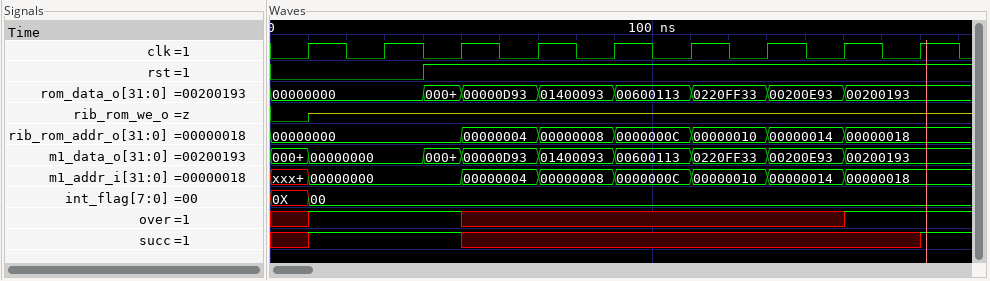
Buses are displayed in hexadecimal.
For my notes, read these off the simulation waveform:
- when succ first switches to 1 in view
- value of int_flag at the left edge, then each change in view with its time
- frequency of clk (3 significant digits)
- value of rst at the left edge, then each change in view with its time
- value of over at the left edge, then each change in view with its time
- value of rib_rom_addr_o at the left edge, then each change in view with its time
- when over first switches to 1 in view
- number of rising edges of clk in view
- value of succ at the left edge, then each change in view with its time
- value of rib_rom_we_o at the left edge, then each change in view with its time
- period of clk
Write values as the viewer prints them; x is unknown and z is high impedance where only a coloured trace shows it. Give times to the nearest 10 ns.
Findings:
10 ns
0X, 00 at 10 ns
50.0 MHz
0, 1 at 40 ns
x, 1 at 10 ns, x at 50 ns, 1 at 150 ns
00000000, 00000004 at 50 ns, 00000008 at 70 ns, 0000000C at 90 ns, 00000010 at 110 ns, 00000014 at 130 ns, 00000018 at 150 ns
10 ns
9
x, 1 at 10 ns, x at 50 ns, 1 at 170 ns
0, z at 10 ns
20 ns
